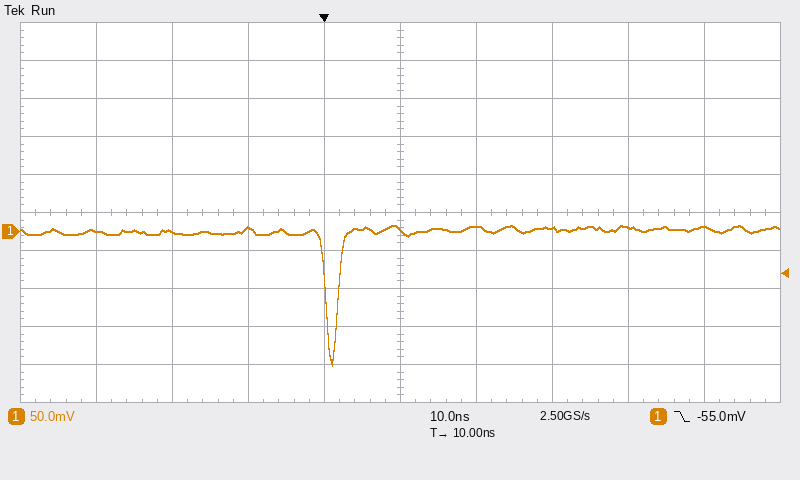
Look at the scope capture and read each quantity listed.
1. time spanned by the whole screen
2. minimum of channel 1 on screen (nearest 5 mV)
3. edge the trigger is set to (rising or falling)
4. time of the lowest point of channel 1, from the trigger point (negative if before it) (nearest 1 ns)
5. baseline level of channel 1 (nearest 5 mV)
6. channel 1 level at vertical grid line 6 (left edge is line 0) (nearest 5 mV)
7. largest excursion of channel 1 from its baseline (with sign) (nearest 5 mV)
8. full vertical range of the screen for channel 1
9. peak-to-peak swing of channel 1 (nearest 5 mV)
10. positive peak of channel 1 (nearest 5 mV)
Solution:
100 ns
-175 mV
falling
+1 ns
0 mV
5 mV
-175 mV
500 mV
185 mV
10 mV
